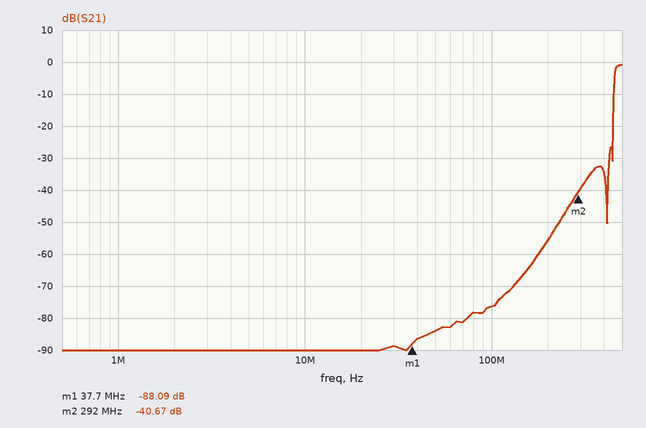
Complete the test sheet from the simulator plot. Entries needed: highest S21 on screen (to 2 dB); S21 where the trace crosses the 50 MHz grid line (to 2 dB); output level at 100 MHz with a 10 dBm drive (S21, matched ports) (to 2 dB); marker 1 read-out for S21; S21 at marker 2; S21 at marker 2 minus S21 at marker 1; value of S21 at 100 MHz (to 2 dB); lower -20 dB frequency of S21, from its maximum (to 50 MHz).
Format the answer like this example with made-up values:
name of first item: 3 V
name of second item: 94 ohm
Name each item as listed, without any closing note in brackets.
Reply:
highest S21 on screen: 0 dB
S21 where the trace crosses the 50 MHz grid line: -84 dB
output level at 100 MHz with a 10 dBm drive (S21, matched ports): -66 dBm
marker 1 read-out for S21: -88.09 dB
S21 at marker 2: -40.67 dB
S21 at marker 2 minus S21 at marker 1: 47.42 dB
value of S21 at 100 MHz: -76 dB
lower -20 dB frequency of S21, from its maximum: 450 MHz
